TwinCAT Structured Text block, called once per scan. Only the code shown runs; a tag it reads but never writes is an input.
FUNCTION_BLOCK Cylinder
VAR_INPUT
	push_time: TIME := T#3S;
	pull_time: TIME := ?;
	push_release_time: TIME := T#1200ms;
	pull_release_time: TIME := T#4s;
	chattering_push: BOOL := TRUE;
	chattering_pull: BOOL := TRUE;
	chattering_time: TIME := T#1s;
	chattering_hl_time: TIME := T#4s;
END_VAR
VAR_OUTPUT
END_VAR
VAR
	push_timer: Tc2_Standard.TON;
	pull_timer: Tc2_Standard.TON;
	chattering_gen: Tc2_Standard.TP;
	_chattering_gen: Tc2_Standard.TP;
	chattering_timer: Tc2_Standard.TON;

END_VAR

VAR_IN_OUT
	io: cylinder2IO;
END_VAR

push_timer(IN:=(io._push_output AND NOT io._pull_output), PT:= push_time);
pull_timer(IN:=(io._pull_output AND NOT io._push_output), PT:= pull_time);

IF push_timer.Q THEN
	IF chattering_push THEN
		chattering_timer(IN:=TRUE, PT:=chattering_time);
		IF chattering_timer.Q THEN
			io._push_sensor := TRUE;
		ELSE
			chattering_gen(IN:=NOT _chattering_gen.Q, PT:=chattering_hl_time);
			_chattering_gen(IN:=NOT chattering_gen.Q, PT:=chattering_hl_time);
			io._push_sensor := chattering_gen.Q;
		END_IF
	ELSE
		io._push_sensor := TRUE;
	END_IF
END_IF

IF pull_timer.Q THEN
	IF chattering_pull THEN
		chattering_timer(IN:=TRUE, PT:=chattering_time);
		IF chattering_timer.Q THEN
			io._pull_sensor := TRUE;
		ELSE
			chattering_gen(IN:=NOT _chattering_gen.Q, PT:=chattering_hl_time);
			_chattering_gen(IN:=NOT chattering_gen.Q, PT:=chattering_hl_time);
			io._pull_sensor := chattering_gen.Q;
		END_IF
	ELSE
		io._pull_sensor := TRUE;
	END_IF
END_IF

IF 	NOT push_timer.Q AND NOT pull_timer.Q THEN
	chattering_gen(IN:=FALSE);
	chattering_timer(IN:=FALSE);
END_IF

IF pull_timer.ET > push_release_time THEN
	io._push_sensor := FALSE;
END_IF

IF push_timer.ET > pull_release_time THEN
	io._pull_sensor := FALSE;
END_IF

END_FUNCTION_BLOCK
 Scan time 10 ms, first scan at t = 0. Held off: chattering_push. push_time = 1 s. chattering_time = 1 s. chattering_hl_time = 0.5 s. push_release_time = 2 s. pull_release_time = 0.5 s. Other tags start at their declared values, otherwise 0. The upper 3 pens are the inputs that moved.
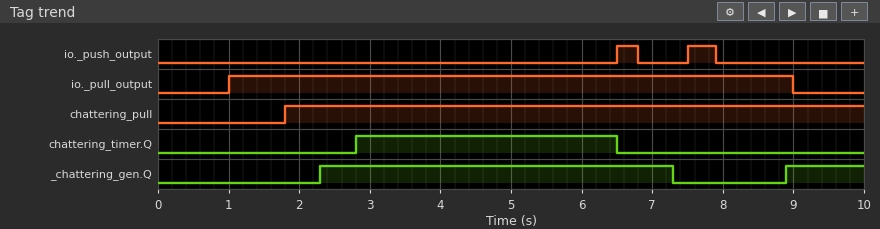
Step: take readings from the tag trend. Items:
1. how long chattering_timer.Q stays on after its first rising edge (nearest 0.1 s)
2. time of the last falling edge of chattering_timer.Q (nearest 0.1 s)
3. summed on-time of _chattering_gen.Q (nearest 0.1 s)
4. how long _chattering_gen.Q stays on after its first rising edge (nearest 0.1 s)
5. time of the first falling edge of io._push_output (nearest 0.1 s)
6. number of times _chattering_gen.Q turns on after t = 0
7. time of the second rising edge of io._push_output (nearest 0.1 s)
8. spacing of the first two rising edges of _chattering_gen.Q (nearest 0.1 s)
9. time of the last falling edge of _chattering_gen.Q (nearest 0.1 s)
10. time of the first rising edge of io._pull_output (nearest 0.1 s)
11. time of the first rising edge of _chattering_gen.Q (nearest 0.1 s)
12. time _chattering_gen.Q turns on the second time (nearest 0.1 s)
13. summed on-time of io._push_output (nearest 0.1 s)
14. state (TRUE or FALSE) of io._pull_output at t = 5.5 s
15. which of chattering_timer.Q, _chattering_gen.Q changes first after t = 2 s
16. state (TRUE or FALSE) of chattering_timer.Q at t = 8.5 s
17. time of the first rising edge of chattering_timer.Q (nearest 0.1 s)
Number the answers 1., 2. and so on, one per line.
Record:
1. 3.7 s
2. 6.5 s
3. 6.1 s
4. 5.0 s
5. 6.8 s
6. 2
7. 7.5 s
8. 6.6 s
9. 7.3 s
10. 1.0 s
11. 2.3 s
12. 8.9 s
13. 0.7 s
14. TRUE
15. _chattering_gen.Q
16. FALSE
17. 2.8 s
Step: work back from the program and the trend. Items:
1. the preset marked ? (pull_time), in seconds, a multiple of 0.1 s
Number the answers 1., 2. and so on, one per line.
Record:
1. 0.5 s
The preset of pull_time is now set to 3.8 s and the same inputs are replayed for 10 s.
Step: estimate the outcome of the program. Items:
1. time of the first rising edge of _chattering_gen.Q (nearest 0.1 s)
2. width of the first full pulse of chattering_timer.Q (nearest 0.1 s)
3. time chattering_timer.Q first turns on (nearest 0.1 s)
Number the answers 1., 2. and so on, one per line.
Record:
1. 5.3 s
2. 0.7 s
3. 5.8 s
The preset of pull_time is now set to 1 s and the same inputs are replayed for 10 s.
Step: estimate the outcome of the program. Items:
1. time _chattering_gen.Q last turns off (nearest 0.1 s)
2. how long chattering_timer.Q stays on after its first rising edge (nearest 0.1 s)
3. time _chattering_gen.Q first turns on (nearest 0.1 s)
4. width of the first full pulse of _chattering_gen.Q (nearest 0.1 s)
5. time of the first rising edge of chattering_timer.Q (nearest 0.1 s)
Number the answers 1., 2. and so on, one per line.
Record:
1. 8.9 s
2. 3.5 s
3. 2.5 s
4. 6.4 s
5. 3.0 s
